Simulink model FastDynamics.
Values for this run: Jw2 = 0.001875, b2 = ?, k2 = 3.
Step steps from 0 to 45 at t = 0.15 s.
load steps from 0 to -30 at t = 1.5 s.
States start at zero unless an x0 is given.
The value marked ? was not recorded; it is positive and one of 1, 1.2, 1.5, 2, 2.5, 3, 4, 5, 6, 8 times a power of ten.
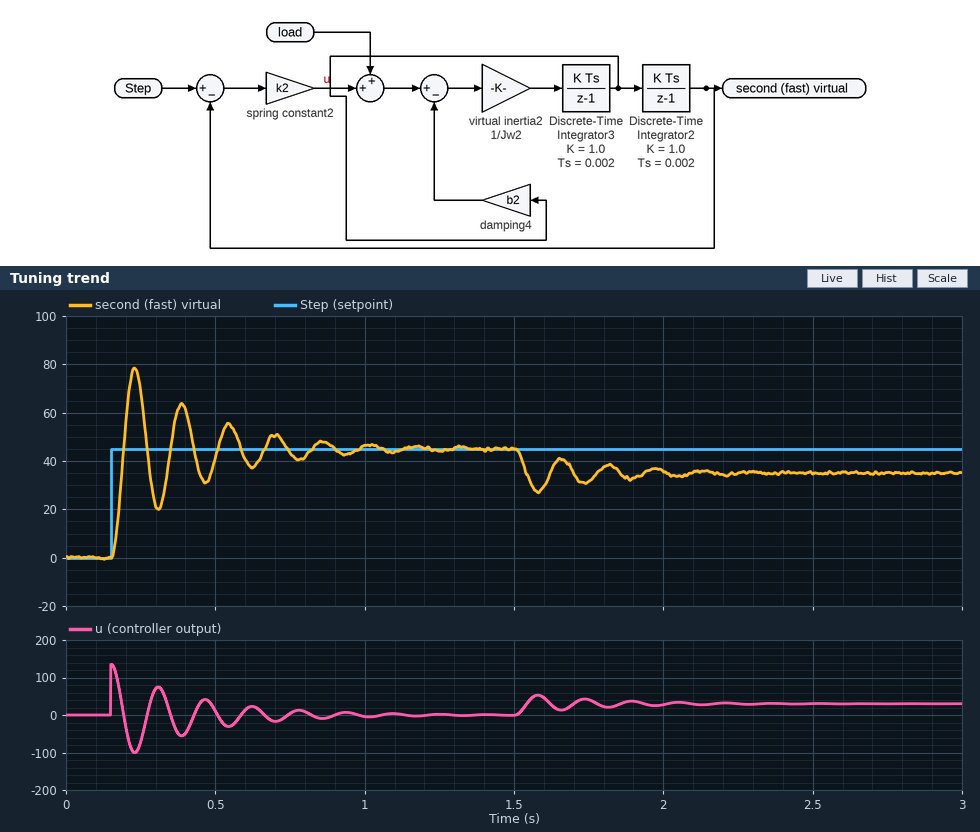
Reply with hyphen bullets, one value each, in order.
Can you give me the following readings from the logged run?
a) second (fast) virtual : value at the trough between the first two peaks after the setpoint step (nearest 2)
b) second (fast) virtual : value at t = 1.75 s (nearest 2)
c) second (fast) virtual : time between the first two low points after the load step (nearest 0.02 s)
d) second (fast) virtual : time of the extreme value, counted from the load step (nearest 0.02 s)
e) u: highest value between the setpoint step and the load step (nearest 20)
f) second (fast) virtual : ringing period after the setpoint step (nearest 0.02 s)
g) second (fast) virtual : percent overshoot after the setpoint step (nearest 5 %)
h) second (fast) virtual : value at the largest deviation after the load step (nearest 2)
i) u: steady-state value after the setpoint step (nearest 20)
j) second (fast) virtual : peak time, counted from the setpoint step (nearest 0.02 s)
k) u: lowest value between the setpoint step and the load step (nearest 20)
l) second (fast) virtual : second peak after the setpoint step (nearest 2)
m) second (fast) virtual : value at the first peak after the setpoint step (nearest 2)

- 20
- 32
- 0.16 s
- 0.08 s
- 140
- 0.16 s
- 75 %
- 28
- 0
- 0.08 s
- -100
- 64
- 78
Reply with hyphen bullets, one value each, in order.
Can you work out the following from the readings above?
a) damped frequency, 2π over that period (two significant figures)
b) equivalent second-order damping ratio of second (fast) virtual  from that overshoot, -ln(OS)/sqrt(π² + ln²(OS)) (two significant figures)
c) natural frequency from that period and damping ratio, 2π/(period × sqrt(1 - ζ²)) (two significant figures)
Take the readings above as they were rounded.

- 39 rad/s
- 0.091
- 39 rad/s
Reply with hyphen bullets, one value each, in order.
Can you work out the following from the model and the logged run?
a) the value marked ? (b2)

- 0.02
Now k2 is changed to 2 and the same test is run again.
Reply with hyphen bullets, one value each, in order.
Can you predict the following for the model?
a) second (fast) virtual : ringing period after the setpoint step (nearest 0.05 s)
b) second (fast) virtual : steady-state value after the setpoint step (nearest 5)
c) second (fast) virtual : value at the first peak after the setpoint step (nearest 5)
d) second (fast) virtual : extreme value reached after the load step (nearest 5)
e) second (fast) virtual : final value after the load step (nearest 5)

- 0.20 s
- 45
- 75
- 20
- 30
